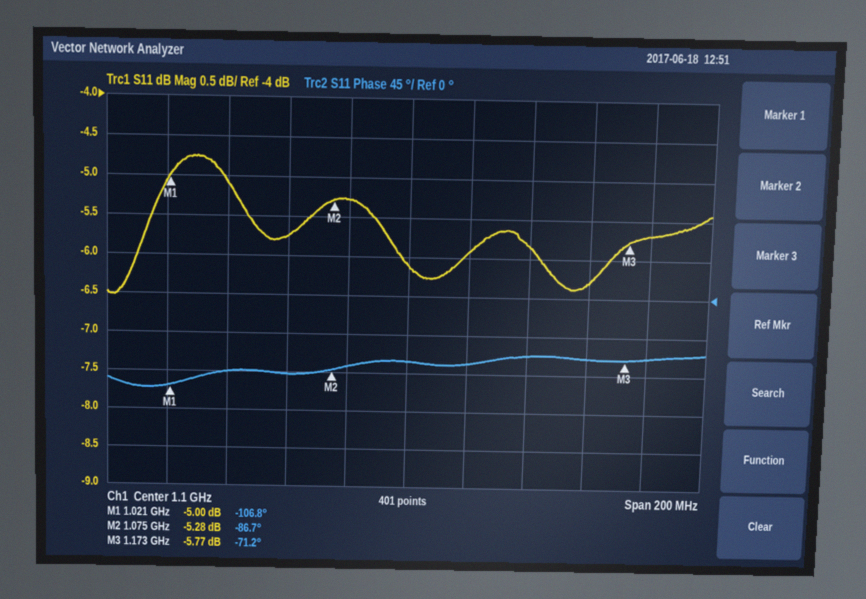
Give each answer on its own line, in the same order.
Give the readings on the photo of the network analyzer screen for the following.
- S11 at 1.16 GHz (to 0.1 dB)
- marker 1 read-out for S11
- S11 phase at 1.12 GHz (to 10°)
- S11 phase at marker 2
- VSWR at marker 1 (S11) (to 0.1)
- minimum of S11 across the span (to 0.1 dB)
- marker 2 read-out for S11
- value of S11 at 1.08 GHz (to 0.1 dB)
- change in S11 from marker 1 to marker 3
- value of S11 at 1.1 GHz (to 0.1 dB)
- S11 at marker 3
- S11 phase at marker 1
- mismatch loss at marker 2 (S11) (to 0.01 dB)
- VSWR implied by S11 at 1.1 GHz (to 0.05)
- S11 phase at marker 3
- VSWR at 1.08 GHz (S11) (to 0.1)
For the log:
-6.3 dB
-5.00 dB
-80°
-86.7°
3.6
-6.5 dB
-5.28 dB
-5.3 dB
-0.77 dB
-6.1 dB
-5.77 dB
-106.8°
1.53 dB
2.95
-71.2°
3.4
